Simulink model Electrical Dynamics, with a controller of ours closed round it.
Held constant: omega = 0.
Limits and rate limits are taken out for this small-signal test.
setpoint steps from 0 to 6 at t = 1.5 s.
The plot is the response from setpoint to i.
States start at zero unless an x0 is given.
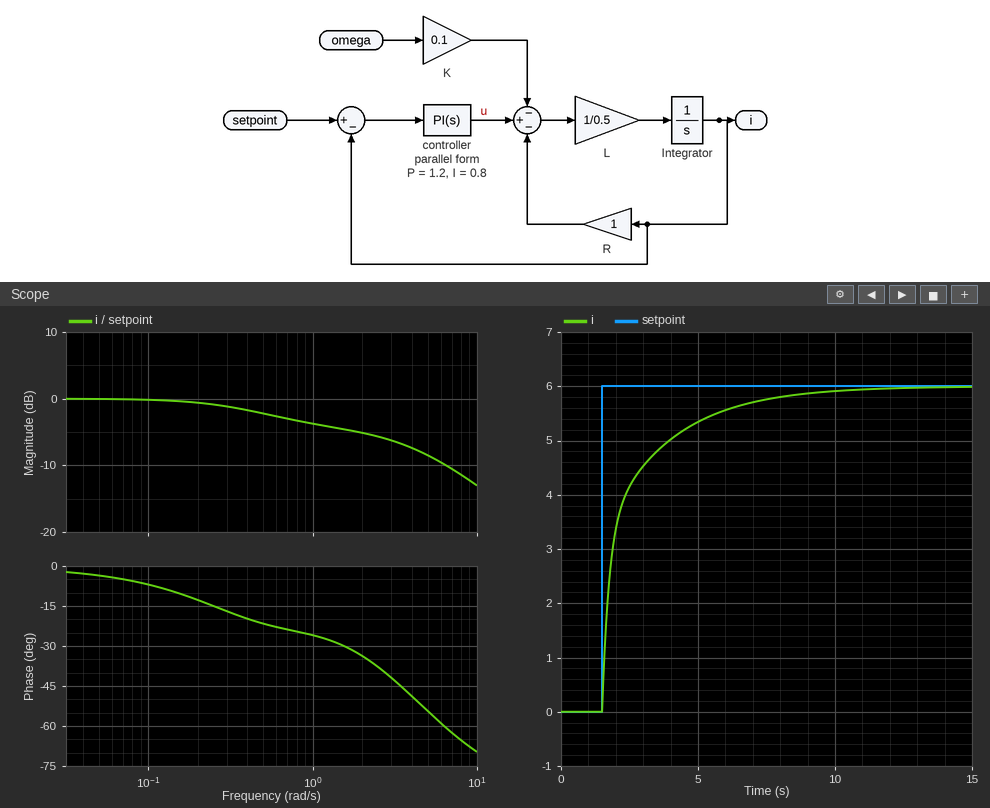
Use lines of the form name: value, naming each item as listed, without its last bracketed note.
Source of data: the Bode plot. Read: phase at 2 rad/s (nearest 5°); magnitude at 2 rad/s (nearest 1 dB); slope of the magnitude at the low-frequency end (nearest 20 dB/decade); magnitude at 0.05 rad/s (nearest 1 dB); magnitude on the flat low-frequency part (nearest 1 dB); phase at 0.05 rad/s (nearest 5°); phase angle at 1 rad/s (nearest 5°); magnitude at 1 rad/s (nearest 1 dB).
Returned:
phase at 2 rad/s: -35°
magnitude at 2 rad/s: -5 dB
slope of the magnitude at the low-frequency end: 0 dB/decade
magnitude at 0.05 rad/s: 0 dB
magnitude on the flat low-frequency part: 0 dB
phase at 0.05 rad/s: -5°
phase angle at 1 rad/s: -25°
magnitude at 1 rad/s: -4 dB
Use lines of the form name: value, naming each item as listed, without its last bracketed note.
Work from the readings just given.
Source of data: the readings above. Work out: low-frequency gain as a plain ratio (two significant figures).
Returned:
low-frequency gain as a plain ratio: 1.0
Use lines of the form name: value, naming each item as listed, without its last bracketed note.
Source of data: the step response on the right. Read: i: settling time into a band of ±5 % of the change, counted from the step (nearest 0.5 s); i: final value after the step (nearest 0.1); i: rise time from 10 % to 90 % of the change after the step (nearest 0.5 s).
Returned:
i: settling time into a band of ±5 % of the change, counted from the step: 5.5 s
i: final value after the step: 6.0
i: rise time from 10 % to 90 % of the change after the step: 3.5 s
